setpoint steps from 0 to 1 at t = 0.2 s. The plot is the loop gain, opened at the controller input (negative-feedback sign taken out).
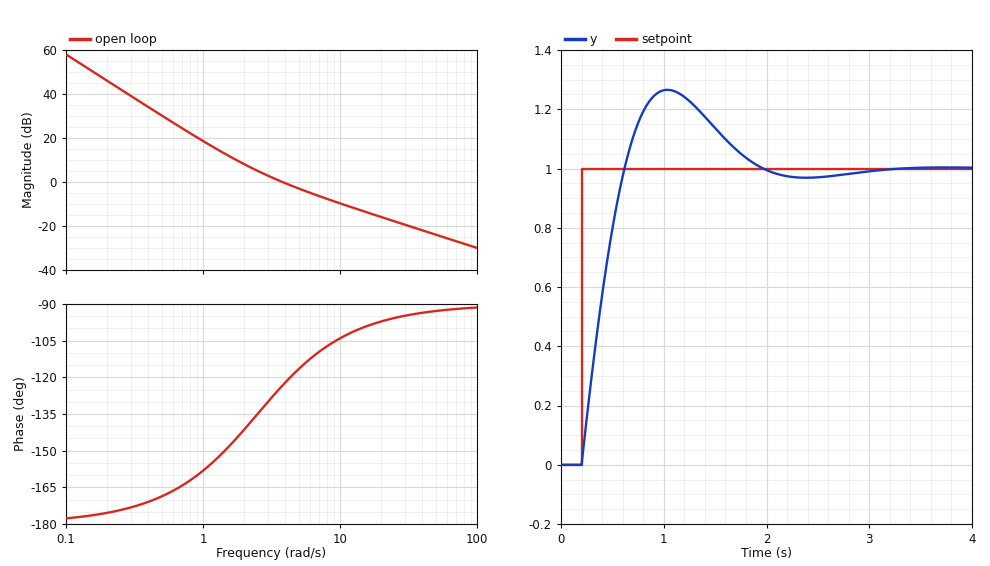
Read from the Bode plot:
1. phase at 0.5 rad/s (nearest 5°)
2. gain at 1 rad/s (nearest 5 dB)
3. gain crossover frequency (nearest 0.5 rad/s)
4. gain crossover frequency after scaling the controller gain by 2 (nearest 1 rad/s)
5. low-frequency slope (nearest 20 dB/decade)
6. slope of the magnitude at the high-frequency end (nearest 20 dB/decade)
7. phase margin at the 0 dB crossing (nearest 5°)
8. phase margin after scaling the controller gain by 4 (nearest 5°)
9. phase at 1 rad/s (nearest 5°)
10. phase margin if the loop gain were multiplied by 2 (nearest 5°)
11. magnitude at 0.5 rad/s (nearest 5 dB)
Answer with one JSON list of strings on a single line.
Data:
["-170°", "20 dB", "4.0 rad/s", "7 rad/s", "-40 dB/decade", "-20 dB/decade", "55°", "80°", "-160°", "70°", "30 dB"]
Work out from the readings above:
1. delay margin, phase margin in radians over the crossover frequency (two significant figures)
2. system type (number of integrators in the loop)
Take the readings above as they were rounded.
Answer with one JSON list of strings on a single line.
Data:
["0.24 s", "2"]
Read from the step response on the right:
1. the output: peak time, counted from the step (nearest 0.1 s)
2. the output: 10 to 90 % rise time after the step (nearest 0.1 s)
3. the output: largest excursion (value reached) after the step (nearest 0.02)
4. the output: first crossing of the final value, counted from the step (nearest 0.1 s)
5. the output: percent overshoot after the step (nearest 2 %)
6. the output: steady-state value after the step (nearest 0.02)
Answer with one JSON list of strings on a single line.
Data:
["0.8 s", "0.3 s", "1.26", "0.4 s", "26 %", "1.00"]
